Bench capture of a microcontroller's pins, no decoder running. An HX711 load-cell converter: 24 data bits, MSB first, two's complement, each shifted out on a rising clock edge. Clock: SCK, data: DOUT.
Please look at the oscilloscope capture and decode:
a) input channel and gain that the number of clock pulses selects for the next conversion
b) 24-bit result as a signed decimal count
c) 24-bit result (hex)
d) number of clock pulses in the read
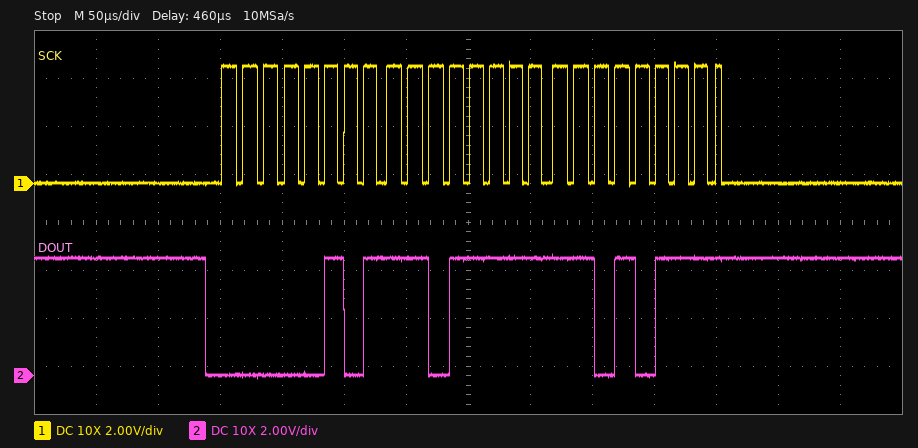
channel A, gain 128
384983
0x05DFD7
25
